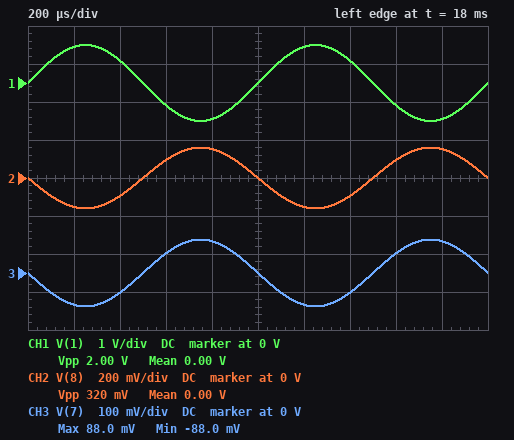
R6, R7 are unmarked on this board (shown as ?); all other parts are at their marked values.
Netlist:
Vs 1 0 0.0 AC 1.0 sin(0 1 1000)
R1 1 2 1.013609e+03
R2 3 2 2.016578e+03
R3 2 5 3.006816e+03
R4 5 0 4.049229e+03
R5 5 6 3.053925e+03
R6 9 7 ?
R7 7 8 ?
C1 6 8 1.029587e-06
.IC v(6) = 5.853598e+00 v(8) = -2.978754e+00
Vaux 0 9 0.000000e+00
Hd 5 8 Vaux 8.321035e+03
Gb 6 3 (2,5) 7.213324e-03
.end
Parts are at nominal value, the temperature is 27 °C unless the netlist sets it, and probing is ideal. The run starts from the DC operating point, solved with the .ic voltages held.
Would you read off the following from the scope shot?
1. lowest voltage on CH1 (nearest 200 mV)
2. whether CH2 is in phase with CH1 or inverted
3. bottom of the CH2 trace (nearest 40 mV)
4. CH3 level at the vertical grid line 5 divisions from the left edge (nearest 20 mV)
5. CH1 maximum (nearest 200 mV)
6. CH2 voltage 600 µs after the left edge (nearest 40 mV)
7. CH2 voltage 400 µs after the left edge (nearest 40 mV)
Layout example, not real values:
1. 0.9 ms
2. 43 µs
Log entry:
1. -1.0 V
2. inverted
3. -160 mV
4. 0 V
5. 1.0 V
6. 80 mV
7. -80 mV
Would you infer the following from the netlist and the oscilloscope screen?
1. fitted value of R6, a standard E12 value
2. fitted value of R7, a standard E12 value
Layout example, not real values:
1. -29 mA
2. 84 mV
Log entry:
1. 680 Ω
2. 560 Ω
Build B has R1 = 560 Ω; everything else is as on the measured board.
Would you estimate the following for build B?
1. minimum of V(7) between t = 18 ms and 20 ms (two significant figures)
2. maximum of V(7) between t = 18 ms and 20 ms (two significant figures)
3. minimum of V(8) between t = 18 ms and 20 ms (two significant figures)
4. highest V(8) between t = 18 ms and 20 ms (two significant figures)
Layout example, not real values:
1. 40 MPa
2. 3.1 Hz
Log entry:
1. -92 mV
2. 92 mV
3. -170 mV
4. 170 mV
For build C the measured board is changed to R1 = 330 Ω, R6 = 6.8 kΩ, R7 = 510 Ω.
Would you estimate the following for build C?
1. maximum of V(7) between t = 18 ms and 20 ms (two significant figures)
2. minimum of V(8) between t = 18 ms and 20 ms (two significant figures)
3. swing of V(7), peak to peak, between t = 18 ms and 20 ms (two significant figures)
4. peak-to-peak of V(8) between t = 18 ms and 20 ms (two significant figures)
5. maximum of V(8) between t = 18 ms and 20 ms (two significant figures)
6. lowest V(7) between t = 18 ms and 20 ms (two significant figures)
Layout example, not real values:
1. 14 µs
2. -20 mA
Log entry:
1. 7.8 V
2. -8.4 V
3. 16 V
4. 17 V
5. 8.4 V
6. -7.8 V
